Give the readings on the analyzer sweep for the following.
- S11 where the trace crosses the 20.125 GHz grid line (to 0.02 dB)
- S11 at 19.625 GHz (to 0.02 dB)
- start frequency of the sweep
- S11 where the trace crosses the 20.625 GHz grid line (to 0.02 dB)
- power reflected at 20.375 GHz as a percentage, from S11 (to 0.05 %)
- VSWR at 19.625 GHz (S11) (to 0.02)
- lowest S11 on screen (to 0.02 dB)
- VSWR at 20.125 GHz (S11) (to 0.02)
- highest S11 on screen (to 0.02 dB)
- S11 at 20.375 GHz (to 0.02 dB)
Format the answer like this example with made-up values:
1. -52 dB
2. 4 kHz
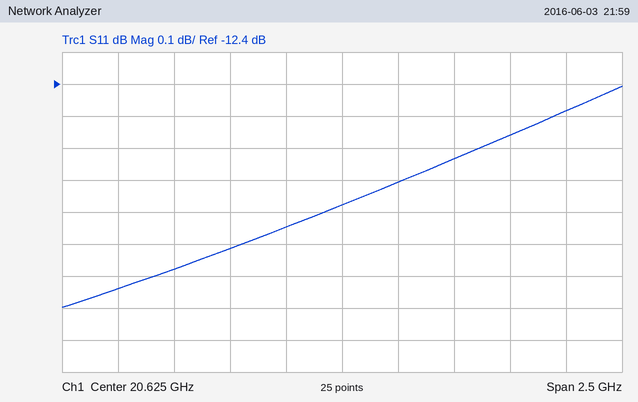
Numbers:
1. -12.92 dB
2. -13.04 dB
3. 19.375 GHz
4. -12.78 dB
5. 5.20 %
6. 1.58
7. -13.10 dB
8. 1.58
9. -12.40 dB
10. -12.84 dB
